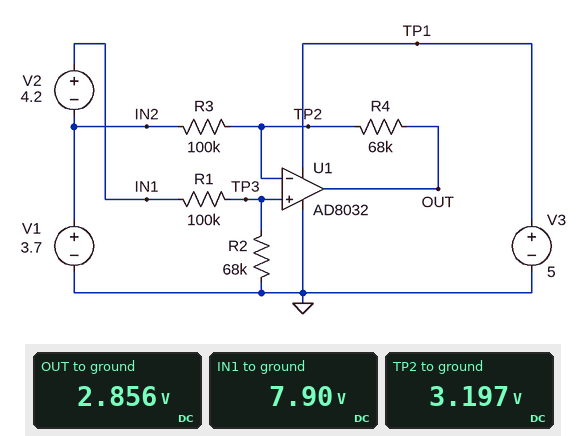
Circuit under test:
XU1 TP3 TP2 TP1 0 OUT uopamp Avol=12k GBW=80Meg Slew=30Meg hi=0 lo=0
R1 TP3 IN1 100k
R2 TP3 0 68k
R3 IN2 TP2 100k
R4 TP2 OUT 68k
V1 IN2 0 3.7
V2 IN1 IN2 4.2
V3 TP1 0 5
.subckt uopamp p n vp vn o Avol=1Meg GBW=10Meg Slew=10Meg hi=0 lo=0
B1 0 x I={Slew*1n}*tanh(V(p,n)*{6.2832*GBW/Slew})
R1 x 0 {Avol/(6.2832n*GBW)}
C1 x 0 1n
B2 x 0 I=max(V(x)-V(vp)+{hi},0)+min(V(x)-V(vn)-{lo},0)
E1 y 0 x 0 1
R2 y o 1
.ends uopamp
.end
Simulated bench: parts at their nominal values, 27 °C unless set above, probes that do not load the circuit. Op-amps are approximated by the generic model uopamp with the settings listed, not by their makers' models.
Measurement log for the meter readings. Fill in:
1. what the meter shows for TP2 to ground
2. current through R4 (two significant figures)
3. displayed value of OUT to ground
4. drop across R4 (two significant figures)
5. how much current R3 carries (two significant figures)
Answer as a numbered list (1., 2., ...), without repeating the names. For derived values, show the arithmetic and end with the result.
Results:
1. 3.197 V
2. (3.197 V - 2.856 V) / 68 kΩ = 5.0 µA
3. 2.856 V
4. 3.197 V - 2.856 V = 340 mV
5. (3.7 V - 3.197 V) / 100 kΩ = 5.0 µA
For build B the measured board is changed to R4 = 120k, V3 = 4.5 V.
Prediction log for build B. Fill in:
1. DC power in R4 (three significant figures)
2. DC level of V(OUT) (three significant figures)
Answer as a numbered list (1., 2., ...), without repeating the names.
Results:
1. 3.03 µW
2. 2.59 V
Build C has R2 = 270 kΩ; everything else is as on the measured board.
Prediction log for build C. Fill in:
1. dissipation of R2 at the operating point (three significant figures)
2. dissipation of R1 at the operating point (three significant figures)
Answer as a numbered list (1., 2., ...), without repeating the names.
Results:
1. 123 µW
2. 45.6 µW
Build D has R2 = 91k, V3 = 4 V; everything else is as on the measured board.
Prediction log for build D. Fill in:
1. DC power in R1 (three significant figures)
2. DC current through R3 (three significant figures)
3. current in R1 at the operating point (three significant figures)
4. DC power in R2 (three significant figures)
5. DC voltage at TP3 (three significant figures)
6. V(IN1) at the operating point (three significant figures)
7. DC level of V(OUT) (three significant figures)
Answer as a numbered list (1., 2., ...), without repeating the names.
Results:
1. 171 µW
2. 636 nA
3. 41.4 µA
4. 156 µW
5. 3.76 V
6. 7.90 V
7. 3.81 V
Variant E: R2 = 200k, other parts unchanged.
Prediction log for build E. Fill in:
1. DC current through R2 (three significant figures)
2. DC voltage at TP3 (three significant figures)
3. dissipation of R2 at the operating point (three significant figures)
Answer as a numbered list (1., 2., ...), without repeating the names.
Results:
1. 26.3 µA
2. 5.27 V
3. 139 µW
